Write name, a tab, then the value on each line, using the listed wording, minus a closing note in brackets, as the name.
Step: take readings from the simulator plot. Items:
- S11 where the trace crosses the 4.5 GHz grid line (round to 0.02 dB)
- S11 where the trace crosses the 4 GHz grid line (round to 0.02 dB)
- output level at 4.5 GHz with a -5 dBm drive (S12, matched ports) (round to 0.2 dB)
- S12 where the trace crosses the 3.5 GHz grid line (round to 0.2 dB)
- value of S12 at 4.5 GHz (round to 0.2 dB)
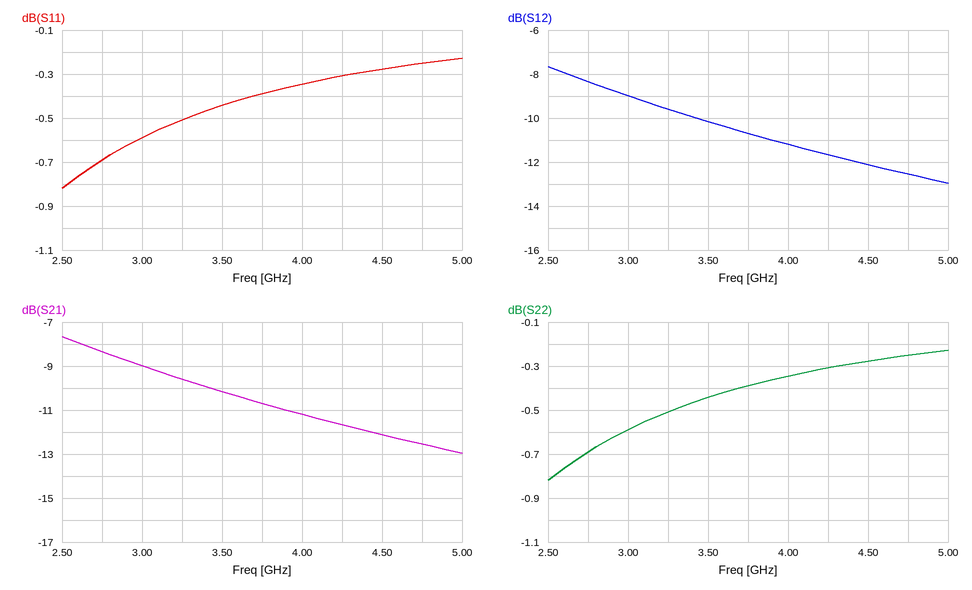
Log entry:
S11 where the trace crosses the 4.5 GHz grid line	-0.28 dB
S11 where the trace crosses the 4 GHz grid line	-0.34 dB
output level at 4.5 GHz with a -5 dBm drive (S12, matched ports)	-17.2 dBm
S12 where the trace crosses the 3.5 GHz grid line	-10.2 dB
value of S12 at 4.5 GHz	-12.2 dB
